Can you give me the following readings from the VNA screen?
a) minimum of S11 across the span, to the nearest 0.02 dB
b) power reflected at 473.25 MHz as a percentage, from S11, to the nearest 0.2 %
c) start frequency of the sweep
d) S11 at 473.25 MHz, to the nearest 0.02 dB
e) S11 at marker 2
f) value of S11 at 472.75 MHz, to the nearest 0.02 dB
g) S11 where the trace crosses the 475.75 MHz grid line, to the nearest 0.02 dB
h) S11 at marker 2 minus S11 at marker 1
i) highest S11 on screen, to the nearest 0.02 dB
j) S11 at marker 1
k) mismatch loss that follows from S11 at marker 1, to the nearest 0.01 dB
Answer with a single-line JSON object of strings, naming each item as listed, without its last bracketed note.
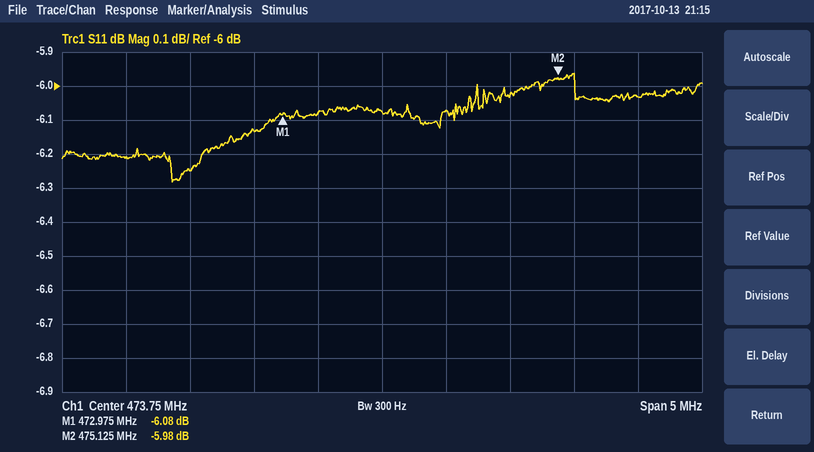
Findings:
{"minimum of S11 across the span, to the nearest 0.02 dB": "-6.28 dB", "power reflected at 473.25 MHz as a percentage, from S11, to the nearest 0.2 %": "24.6 %", "start frequency of the sweep": "471.25 MHz", "S11 at 473.25 MHz, to the nearest 0.02 dB": "-6.08 dB", "S11 at marker 2": "-5.98 dB", "value of S11 at 472.75 MHz, to the nearest 0.02 dB": "-6.14 dB", "S11 where the trace crosses the 475.75 MHz grid line, to the nearest 0.02 dB": "-6.04 dB", "S11 at marker 2 minus S11 at marker 1": "0.10 dB", "highest S11 on screen, to the nearest 0.02 dB": "-5.96 dB", "S11 at marker 1": "-6.08 dB", "mismatch loss that follows from S11 at marker 1, to the nearest 0.01 dB": "1.23 dB"}
